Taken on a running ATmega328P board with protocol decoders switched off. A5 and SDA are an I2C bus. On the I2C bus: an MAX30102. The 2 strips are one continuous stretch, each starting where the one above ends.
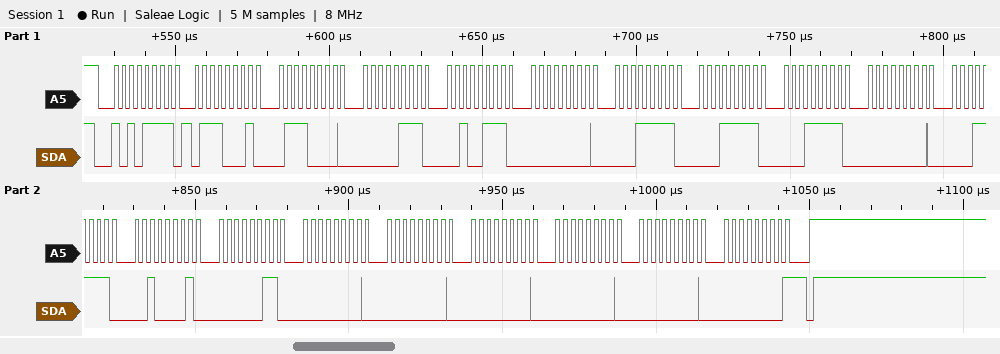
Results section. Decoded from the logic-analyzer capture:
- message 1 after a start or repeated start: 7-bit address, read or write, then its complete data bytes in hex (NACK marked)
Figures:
0x57 read: 71 70 07 27 00 1F 1F 1F 00 1F 21 03 00 00 00 00 00 00 NACK
